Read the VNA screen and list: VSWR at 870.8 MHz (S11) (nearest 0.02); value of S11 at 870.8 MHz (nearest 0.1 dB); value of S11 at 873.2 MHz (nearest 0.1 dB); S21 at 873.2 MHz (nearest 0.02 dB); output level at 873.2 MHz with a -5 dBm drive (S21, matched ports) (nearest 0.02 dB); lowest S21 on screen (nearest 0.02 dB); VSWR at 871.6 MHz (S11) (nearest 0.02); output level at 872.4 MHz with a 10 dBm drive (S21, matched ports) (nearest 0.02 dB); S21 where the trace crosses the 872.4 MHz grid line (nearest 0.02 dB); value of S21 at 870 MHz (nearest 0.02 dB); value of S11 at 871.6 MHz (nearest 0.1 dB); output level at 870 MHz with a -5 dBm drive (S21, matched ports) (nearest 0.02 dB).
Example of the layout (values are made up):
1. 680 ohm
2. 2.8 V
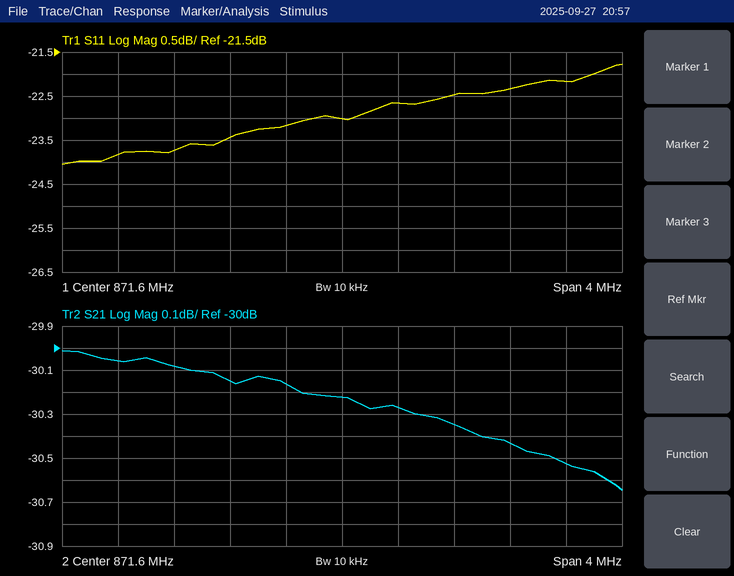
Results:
1. 1.14
2. -23.4 dB
3. -22.2 dB
4. -30.52 dB
5. -35.52 dBm
6. -30.64 dB
7. 1.16
8. -20.34 dBm
9. -30.34 dB
10. -30.06 dB
11. -23.0 dB
12. -35.06 dBm
